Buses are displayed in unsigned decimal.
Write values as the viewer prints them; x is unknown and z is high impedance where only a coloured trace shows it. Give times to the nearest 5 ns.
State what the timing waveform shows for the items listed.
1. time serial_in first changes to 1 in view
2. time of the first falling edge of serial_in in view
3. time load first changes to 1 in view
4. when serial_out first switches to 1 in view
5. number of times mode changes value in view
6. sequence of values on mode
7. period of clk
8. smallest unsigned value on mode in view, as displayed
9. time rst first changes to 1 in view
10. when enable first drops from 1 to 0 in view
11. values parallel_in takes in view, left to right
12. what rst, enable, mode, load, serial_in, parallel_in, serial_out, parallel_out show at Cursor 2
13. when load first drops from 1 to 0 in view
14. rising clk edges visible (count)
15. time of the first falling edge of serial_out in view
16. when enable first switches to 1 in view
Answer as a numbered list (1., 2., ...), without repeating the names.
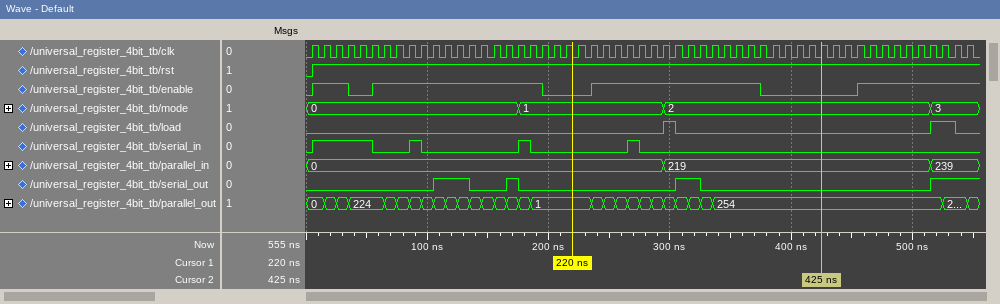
1. 5 ns
2. 55 ns
3. 295 ns
4. 105 ns
5. 3
6. 0, 1, 2, 3
7. 10 ns
8. 0
9. 5 ns
10. 35 ns
11. 0, 219, 239
12. rst=1, enable=0, mode=2, load=0, serial_in=0, parallel_in=219, serial_out=0, parallel_out=254
13. 305 ns
14. 55
15. 135 ns
16. 5 ns
